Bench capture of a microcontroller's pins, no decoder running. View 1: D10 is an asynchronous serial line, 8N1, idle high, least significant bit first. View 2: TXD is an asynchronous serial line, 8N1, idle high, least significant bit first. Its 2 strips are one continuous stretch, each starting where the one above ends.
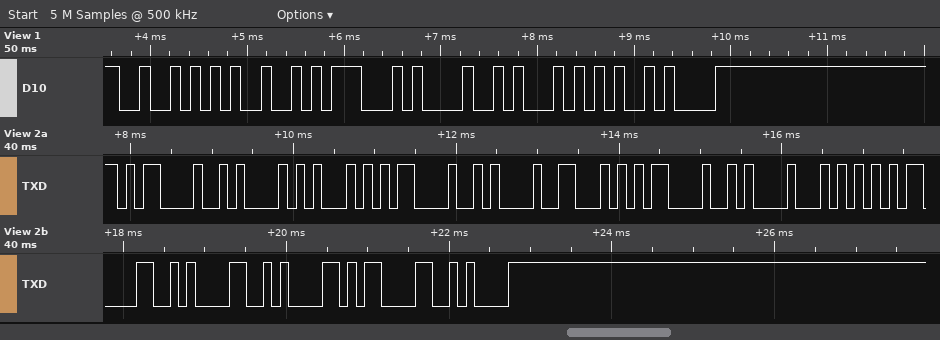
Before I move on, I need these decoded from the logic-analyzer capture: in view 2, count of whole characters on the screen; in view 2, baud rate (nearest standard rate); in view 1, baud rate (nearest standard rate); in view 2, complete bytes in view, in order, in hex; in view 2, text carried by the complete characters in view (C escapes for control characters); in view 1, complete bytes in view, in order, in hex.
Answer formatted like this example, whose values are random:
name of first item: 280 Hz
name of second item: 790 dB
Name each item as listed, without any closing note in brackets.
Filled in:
in view 2, count of whole characters on the screen: 14
in view 2, baud rate: 9600 baud
in view 1, baud rate: 9600 baud
in view 2, complete bytes in view, in order, in hex: 0x0D 0x0A 0x45 0x0D 0x0A 0x46 0x0D 0x0A 0x54 0x0D 0x0A 0x0A 0x0D 0x0A
in view 2, text carried by the complete characters in view: "\r\nE\r\nF\r\nT\r\n\n\r\n"
in view 1, complete bytes in view, in order, in hex: 52 49 47 48 54 0A
